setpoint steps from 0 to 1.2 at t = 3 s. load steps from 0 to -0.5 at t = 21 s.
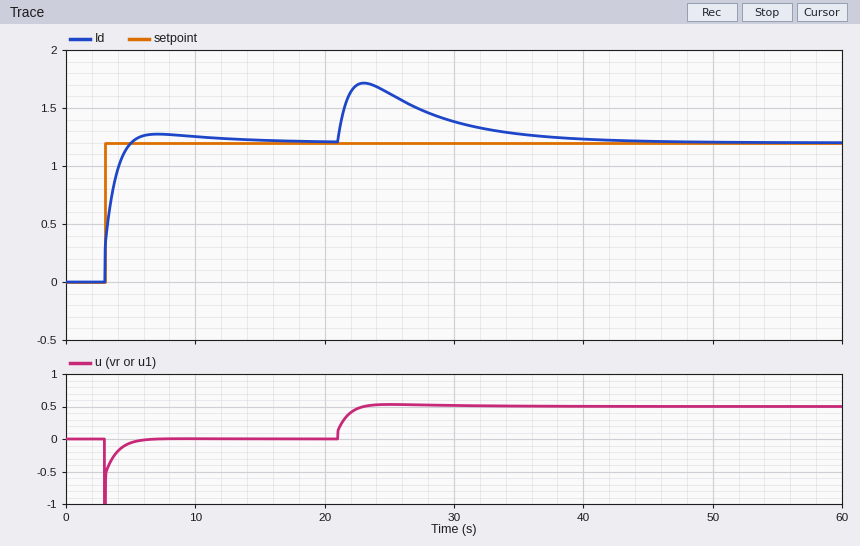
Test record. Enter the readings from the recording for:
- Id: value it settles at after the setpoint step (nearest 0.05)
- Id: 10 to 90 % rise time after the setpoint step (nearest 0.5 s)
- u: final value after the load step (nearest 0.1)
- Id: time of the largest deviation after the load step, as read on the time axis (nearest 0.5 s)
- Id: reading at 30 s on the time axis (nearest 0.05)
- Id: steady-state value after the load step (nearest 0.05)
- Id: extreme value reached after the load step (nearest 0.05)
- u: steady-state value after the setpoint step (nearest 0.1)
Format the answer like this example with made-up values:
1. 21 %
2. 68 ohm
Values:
1. 1.20
2. 1.5 s
3. 0.5
4. 23.0 s
5. 1.40
6. 1.20
7. 1.70
8. 0.0
